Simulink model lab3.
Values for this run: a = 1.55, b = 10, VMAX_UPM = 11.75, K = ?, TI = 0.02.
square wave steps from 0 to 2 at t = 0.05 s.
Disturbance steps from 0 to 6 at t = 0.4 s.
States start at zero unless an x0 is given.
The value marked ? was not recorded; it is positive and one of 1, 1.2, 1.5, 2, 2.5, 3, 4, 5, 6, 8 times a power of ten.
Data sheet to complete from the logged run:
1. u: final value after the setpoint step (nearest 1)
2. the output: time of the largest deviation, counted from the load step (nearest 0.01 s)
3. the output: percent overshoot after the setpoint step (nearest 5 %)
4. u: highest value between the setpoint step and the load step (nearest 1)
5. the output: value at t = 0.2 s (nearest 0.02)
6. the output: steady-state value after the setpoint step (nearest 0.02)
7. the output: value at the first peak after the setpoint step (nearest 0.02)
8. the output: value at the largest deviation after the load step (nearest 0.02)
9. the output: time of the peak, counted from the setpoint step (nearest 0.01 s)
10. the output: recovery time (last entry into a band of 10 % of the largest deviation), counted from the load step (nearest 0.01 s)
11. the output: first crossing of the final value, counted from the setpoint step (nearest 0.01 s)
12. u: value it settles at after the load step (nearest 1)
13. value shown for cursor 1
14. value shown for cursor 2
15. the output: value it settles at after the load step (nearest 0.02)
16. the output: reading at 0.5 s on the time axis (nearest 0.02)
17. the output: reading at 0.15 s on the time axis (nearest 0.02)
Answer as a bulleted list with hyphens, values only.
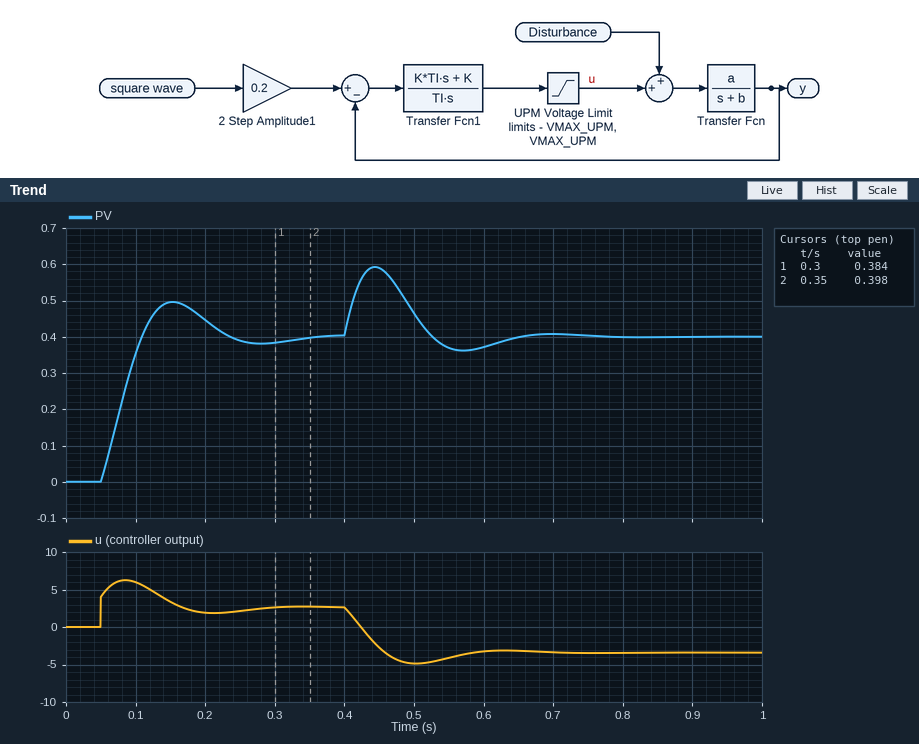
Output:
- 3
- 0.04 s
- 25 %
- 6
- 0.44
- 0.40
- 0.50
- 0.60
- 0.10 s
- 0.22 s
- 0.06 s
- -3
- 0.384
- 0.398
- 0.40
- 0.46
- 0.50
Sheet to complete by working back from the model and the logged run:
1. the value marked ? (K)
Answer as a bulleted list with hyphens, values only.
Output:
- 10
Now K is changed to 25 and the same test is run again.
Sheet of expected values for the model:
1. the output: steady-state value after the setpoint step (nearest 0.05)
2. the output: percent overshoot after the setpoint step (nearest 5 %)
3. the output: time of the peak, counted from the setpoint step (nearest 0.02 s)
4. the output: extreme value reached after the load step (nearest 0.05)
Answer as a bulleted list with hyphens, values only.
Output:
- 0.40
- 20 %
- 0.06 s
- 0.50
